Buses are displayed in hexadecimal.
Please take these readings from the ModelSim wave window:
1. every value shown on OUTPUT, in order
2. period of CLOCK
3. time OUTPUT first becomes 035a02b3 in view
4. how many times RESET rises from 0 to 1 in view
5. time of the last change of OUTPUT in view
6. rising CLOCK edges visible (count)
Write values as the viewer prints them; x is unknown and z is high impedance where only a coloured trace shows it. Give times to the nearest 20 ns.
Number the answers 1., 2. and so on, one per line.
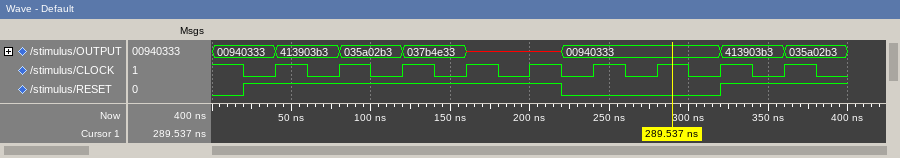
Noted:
1. 00940333, 413903b3, 035a02b3, 037b4e33, x, 00940333, 413903b3, 035a02b3
2. 40 ns
3. 80 ns
4. 2
5. 360 ns
6. 9
